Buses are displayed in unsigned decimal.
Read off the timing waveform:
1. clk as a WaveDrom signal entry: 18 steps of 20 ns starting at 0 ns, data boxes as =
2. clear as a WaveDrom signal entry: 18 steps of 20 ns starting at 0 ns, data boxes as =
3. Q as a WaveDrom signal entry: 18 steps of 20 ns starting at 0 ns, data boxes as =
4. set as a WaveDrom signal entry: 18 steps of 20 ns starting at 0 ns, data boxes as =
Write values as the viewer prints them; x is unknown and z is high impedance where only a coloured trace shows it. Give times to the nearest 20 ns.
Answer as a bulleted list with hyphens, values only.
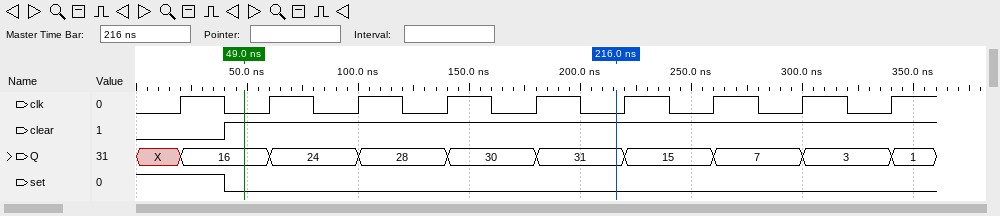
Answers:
- {name: 'clk', wave: '010101010101010101'}
- {name: 'clear', wave: '0.1...............'}
- {name: 'Q', wave: 'x=.=.=.=.=.=.=.=.=', data: '16 24 28 30 31 15 7 3 1'}
- {name: 'set', wave: '1.0...............'}
